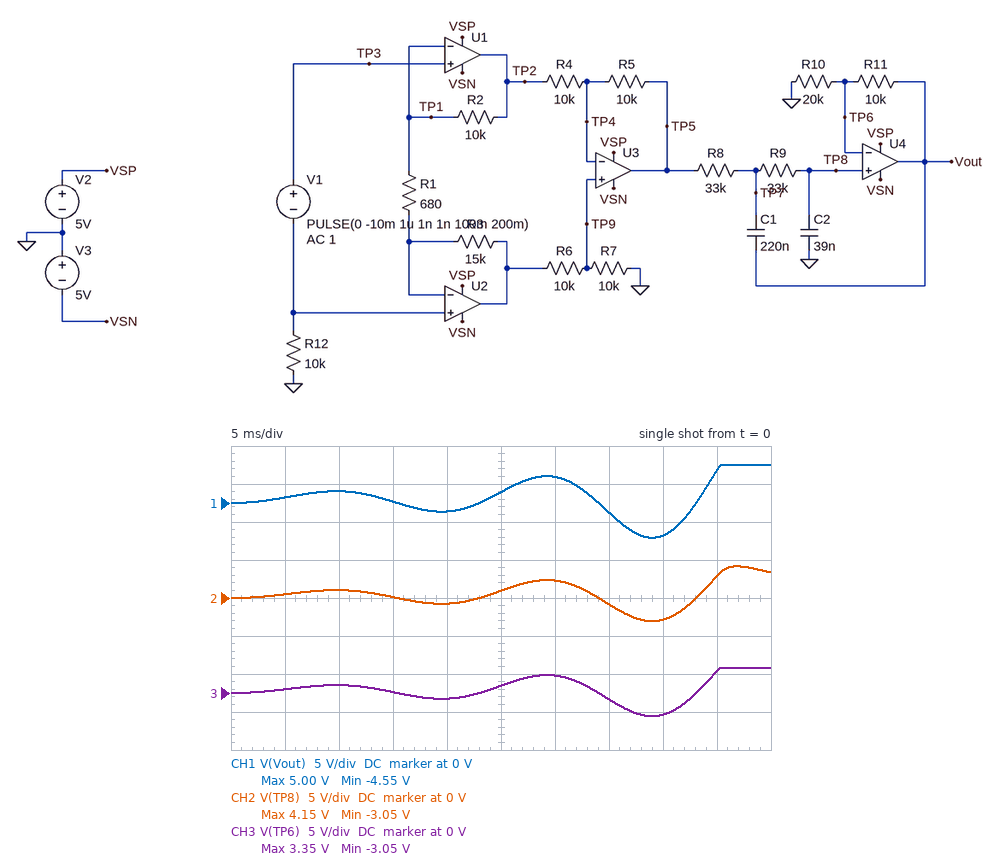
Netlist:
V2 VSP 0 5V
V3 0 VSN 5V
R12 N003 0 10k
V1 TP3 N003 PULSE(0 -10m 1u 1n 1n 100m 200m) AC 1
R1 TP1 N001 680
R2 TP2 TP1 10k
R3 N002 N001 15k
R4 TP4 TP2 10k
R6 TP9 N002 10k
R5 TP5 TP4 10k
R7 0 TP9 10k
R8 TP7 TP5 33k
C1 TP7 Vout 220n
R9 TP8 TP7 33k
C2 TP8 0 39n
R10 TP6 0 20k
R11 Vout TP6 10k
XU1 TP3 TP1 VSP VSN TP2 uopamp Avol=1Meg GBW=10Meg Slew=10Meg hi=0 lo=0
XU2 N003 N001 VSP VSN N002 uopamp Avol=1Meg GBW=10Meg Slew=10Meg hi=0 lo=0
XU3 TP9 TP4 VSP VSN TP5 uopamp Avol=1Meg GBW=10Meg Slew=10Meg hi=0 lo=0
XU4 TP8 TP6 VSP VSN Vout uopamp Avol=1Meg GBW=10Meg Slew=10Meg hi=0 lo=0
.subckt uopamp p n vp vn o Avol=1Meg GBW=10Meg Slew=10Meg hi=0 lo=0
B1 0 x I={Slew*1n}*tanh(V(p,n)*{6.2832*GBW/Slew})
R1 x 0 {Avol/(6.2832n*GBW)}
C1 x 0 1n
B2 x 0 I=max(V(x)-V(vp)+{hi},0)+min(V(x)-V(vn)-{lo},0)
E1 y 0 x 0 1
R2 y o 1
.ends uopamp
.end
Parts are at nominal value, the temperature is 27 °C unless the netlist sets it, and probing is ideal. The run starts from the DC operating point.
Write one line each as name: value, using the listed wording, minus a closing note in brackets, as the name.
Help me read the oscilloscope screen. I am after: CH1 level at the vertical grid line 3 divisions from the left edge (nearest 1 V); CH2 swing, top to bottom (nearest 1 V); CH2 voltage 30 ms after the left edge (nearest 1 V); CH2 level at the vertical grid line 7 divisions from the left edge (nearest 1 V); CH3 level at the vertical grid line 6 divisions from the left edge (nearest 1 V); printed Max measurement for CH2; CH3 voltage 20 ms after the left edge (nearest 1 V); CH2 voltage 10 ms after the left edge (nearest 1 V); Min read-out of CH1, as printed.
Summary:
CH1 level at the vertical grid line 3 divisions from the left edge: 0 V
CH2 swing, top to bottom: 7 V
CH2 voltage 30 ms after the left edge: 2 V
CH2 level at the vertical grid line 7 divisions from the left edge: -1 V
CH3 level at the vertical grid line 6 divisions from the left edge: 2 V
printed Max measurement for CH2: 4.15 V
CH3 voltage 20 ms after the left edge: -1 V
CH2 voltage 10 ms after the left edge: 1 V
Min read-out of CH1, as printed: -4.55 V
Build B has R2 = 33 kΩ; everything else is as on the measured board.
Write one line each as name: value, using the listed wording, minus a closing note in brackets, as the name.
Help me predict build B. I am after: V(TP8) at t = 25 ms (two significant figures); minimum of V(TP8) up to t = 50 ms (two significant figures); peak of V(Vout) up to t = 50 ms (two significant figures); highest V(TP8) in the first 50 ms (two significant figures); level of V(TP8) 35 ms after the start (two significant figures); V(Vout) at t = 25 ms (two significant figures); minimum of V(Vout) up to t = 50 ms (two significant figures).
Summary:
V(TP8) at t = 25 ms: 1.8 V
minimum of V(TP8) up to t = 50 ms: -3.6 V
peak of V(Vout) up to t = 50 ms: 5.0 V
highest V(TP8) in the first 50 ms: 4.5 V
level of V(TP8) 35 ms after the start: -970 mV
V(Vout) at t = 25 ms: 2.7 V
minimum of V(Vout) up to t = 50 ms: -5.0 V
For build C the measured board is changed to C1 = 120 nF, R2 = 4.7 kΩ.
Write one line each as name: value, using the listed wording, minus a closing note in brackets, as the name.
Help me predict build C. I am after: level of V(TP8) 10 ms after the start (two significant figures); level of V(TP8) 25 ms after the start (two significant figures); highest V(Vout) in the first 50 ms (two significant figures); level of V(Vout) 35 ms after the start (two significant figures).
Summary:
level of V(TP8) 10 ms after the start: 370 mV
level of V(TP8) 25 ms after the start: 310 mV
highest V(Vout) in the first 50 ms: 750 mV
level of V(Vout) 35 ms after the start: 500 mV
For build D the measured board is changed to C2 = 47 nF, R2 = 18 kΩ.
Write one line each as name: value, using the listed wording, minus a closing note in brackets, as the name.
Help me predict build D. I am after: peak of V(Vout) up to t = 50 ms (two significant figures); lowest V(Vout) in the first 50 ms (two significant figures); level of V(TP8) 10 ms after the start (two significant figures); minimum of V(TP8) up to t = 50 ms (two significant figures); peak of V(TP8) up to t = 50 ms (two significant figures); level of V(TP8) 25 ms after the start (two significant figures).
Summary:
peak of V(Vout) up to t = 50 ms: 2.5 V
lowest V(Vout) in the first 50 ms: -1.3 V
level of V(TP8) 10 ms after the start: 1.1 V
minimum of V(TP8) up to t = 50 ms: -840 mV
peak of V(TP8) up to t = 50 ms: 1.6 V
level of V(TP8) 25 ms after the start: 190 mV
